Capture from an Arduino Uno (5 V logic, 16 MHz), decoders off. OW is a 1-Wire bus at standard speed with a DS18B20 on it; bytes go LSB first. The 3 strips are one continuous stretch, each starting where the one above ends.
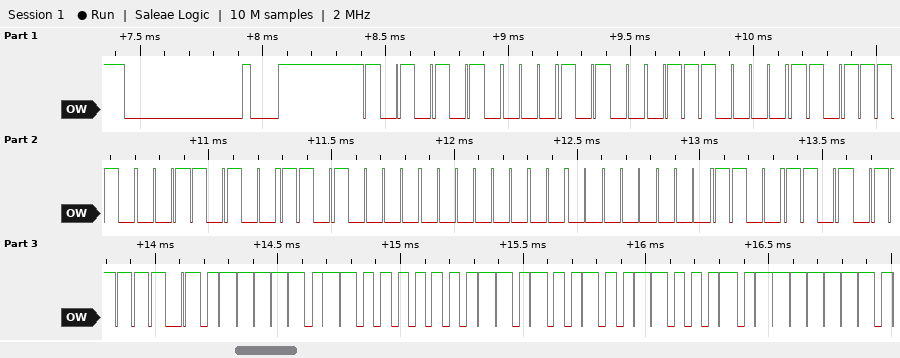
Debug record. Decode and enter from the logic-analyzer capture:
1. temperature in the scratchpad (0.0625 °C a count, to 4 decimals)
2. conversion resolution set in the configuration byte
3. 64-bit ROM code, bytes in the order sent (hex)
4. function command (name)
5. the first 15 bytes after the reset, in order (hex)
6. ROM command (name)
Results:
27.8750 °C
12 bits
28 0E 7B 2C 0B 00 00 B3
Read Scratchpad
55 28 0E 7B 2C 0B 00 00 B3 BE BE 01 4B 46 7F
Match ROM
